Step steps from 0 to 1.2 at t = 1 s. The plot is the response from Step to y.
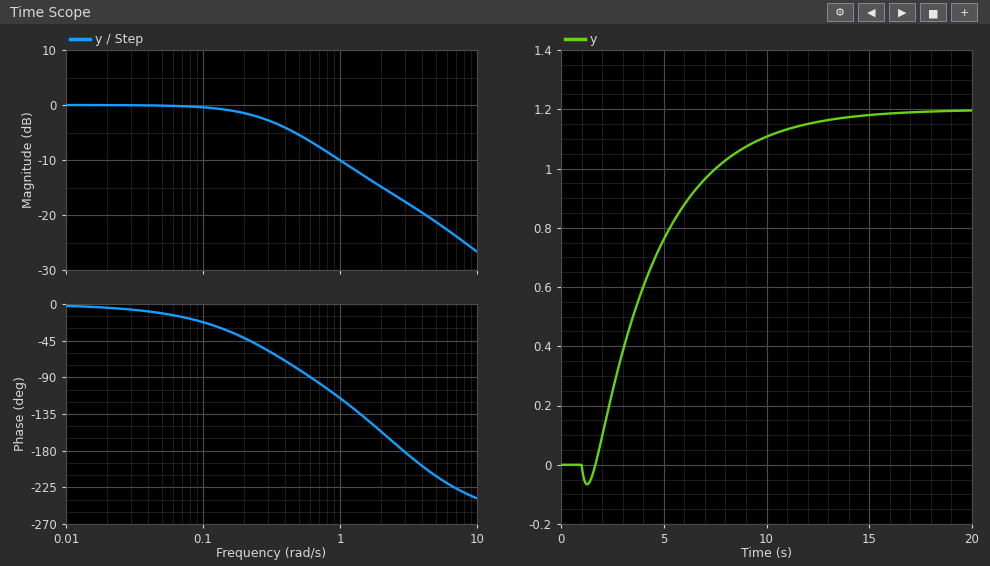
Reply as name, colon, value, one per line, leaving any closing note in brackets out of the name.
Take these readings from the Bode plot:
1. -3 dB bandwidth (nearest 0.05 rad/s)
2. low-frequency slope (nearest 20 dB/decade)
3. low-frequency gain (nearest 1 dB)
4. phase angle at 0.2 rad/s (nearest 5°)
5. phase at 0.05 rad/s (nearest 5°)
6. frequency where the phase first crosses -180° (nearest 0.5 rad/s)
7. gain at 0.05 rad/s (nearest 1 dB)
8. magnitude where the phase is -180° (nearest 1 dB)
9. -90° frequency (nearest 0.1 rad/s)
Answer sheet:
-3 dB bandwidth: 0.30 rad/s
low-frequency slope: 0 dB/decade
low-frequency gain: 0 dB
phase angle at 0.2 rad/s: -40°
phase at 0.05 rad/s: -10°
frequency where the phase first crosses -180°: 3.0 rad/s
gain at 0.05 rad/s: 0 dB
magnitude where the phase is -180°: -17 dB
-90° frequency: 0.6 rad/s
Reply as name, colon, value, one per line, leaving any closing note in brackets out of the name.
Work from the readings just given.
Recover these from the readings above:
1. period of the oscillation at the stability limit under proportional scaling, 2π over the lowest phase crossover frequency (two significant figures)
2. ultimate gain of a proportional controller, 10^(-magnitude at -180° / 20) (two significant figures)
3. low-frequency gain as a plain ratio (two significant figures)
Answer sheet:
period of the oscillation at the stability limit under proportional scaling, 2π over the lowest phase crossover frequency: 2.1 s
ultimate gain of a proportional controller, 10^(-magnitude at -180° / 20): 7.1
low-frequency gain as a plain ratio: 1.0
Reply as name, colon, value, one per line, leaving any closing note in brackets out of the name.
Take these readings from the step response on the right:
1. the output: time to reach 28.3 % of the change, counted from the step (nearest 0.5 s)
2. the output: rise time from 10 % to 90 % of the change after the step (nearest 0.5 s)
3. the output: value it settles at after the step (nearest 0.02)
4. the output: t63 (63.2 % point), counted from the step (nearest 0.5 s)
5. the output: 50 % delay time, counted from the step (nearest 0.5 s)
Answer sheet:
the output: time to reach 28.3 % of the change, counted from the step: 2.0 s
the output: rise time from 10 % to 90 % of the change after the step: 7.0 s
the output: value it settles at after the step: 1.20
the output: t63 (63.2 % point), counted from the step: 4.0 s
the output: 50 % delay time, counted from the step: 3.0 s
